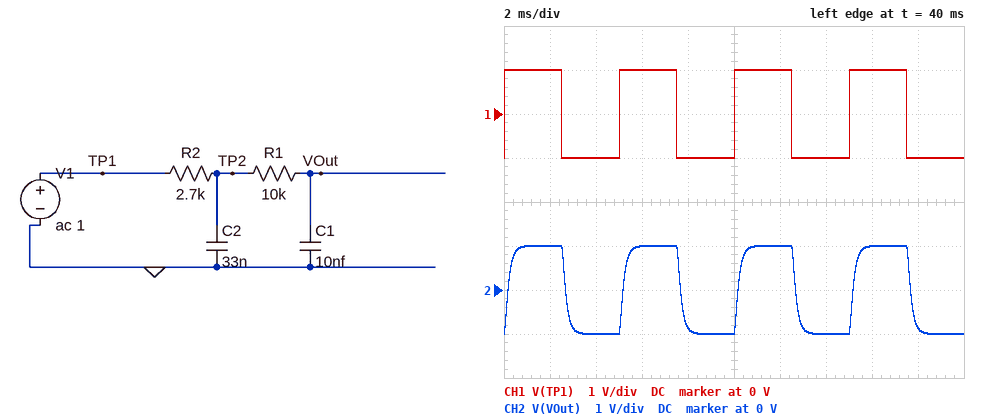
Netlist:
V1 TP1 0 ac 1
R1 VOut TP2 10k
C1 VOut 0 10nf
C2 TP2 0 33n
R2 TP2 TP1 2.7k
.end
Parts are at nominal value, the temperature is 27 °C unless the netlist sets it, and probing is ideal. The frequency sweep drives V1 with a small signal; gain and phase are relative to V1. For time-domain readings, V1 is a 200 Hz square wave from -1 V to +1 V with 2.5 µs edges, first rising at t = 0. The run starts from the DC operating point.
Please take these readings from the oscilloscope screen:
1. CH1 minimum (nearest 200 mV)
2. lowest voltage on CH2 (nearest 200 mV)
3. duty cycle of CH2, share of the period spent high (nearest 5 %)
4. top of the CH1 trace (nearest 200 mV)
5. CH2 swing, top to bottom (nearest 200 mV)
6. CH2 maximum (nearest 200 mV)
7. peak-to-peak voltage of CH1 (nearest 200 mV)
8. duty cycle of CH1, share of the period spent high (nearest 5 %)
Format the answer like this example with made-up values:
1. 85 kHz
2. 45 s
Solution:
1. -1.0 V
2. -1.0 V
3. 50 %
4. 1.0 V
5. 2.0 V
6. 1.0 V
7. 2.0 V
8. 50 %
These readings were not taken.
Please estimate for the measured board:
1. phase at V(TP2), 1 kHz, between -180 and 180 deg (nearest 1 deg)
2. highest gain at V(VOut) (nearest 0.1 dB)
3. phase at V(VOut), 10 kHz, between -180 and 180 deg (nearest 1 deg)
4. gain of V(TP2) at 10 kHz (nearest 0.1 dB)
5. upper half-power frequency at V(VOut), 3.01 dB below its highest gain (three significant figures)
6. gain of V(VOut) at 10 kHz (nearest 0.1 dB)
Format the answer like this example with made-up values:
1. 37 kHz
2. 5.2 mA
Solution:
1. -32 deg
2. 0 dB
3. -158 deg
4. -15.2 dB
5. 898 Hz
6. -31.3 dB
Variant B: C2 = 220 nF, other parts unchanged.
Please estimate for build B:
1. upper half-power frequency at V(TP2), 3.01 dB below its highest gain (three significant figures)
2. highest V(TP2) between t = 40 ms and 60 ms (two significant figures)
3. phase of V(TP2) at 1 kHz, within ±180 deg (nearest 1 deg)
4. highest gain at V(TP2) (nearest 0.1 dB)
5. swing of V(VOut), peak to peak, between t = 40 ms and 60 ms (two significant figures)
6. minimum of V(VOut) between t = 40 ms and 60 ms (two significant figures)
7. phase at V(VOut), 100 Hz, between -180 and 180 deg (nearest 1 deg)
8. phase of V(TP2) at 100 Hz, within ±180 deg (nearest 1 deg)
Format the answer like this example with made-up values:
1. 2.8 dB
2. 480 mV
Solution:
1. 255 Hz
2. 960 mV
3. -74 deg
4. 0 dB
5. 1.9 V
6. -960 mV
7. -25 deg
8. -21 deg
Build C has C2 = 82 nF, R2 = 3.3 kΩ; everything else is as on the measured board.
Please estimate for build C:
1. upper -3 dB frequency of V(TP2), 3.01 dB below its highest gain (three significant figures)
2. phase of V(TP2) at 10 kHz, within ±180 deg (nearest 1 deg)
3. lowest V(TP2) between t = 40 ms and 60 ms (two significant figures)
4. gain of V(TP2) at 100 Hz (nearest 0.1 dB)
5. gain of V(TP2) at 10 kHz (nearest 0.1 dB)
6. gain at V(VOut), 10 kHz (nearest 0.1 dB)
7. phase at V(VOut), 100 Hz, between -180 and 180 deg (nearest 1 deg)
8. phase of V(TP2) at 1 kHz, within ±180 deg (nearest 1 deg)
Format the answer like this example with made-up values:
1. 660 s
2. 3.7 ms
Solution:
1. 513 Hz
2. -86 deg
3. -1.0 V
4. -0.2 dB
5. -24.7 dB
6. -40.7 dB
7. -14 deg
8. -59 deg
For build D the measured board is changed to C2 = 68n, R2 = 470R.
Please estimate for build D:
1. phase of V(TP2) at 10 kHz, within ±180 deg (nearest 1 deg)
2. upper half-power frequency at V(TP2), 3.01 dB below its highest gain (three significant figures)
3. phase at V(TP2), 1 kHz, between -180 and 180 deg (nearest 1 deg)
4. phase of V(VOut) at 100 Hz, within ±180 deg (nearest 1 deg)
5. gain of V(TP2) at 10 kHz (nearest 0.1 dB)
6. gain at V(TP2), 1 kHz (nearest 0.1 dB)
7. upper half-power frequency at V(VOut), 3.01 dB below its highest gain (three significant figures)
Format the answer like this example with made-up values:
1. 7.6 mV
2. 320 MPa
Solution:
1. -63 deg
2. 4.69 kHz
3. -12 deg
4. -5 deg
5. -7.1 dB
6. -0.3 dB
7. 1.39 kHz
